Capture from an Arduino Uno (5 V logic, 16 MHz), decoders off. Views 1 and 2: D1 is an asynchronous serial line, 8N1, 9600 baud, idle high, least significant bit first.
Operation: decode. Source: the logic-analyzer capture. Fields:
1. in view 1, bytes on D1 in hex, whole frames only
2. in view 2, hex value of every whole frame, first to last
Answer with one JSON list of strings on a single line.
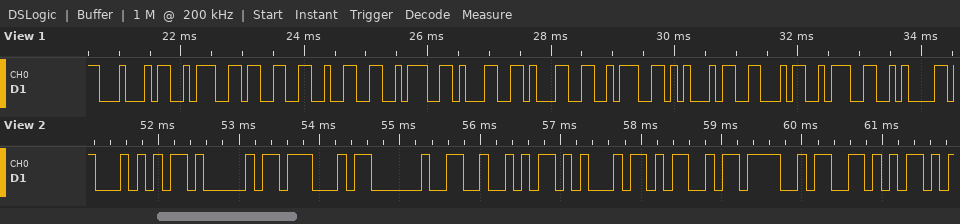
["44 3A 33 32 3A 31 31 3A 45 46 3A 0A", "0x54 0x41 0x47 0x20 0x52 0x45 0x4D 0x4F 0x56"]
